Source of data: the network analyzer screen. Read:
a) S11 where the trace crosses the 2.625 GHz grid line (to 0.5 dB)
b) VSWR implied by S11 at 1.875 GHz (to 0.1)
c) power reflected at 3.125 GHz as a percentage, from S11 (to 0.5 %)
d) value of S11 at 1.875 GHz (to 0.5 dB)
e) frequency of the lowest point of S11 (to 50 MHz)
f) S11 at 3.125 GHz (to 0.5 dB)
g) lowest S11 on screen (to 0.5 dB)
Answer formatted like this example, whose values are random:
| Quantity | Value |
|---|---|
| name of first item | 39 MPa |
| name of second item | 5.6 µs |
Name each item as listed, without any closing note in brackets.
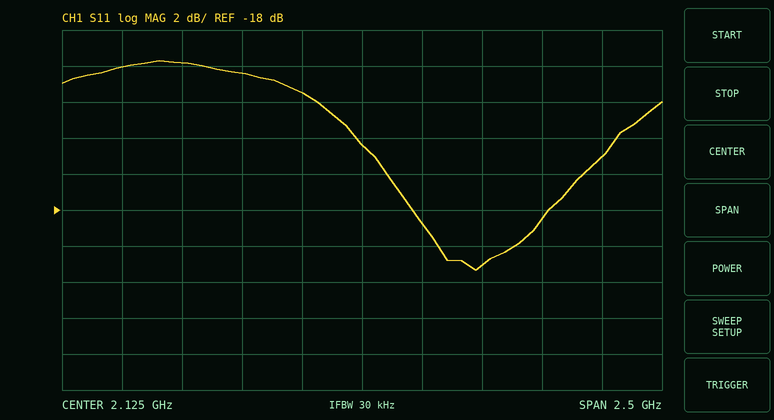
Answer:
| Quantity | Value |
|---|---|
| S11 where the trace crosses the 2.625 GHz grid line | -21.0 dB |
| VSWR implied by S11 at 1.875 GHz | 1.7 |
| power reflected at 3.125 GHz as a percentage, from S11 | 3.0 % |
| value of S11 at 1.875 GHz | -11.5 dB |
| frequency of the lowest point of S11 | 2.60 GHz |
| S11 at 3.125 GHz | -15.0 dB |
| lowest S11 on screen | -21.5 dB |
